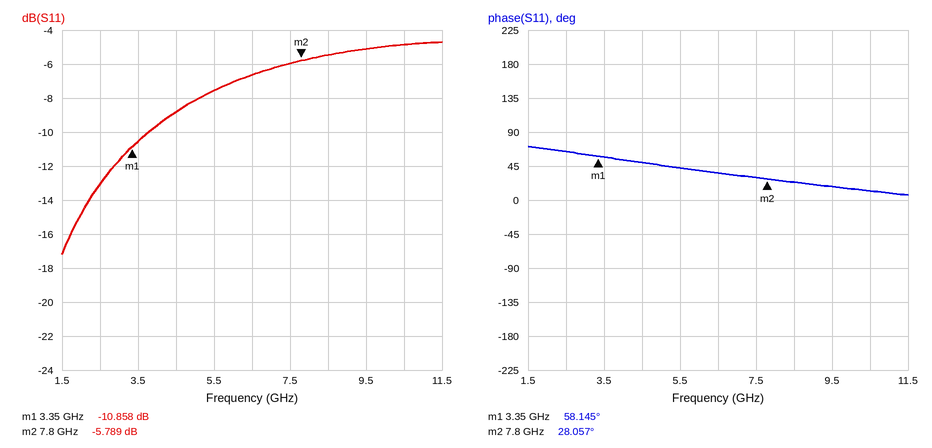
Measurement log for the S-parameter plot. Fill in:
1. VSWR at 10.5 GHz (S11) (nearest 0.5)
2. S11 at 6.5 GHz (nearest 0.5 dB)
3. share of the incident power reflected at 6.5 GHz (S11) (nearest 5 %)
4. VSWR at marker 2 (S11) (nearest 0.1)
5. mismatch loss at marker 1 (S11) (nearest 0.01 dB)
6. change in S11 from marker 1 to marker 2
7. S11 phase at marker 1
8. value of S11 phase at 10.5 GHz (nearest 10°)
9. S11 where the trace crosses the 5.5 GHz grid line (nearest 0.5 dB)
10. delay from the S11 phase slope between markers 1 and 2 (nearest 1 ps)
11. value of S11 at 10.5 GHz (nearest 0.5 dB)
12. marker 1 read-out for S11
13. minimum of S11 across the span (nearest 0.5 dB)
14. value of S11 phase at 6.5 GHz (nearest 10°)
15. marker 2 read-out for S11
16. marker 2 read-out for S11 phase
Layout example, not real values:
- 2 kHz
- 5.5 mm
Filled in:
- 3.5
- -6.5 dB
- 20 %
- 3.1
- 0.37 dB
- 5.069 dB
- 58.145°
- 10°
- -7.5 dB
- 19 ps
- -5.0 dB
- -10.858 dB
- -17.0 dB
- 40°
- -5.789 dB
- 28.057°
